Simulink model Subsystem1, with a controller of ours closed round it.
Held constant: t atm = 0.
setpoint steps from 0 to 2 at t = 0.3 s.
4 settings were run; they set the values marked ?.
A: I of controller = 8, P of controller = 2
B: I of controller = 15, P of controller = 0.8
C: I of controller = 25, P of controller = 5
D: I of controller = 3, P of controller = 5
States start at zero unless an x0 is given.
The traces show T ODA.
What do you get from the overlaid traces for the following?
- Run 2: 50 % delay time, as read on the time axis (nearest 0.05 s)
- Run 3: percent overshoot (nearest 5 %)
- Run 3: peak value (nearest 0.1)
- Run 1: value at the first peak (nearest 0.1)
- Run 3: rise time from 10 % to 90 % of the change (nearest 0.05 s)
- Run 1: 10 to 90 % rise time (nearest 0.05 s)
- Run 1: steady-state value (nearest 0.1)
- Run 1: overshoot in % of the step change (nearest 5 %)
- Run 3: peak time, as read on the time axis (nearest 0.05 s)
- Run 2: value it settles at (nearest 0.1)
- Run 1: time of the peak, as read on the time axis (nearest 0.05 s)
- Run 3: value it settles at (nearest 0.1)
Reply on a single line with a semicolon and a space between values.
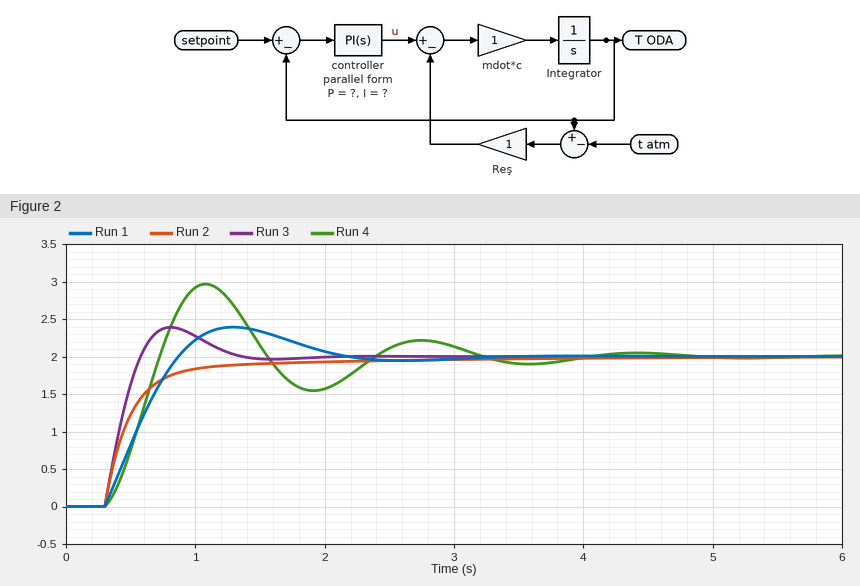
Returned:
0.45 s; 20 %; 2.4; 2.4; 0.20 s; 0.45 s; 2.0; 20 %; 0.80 s; 2.0; 1.30 s; 2.0
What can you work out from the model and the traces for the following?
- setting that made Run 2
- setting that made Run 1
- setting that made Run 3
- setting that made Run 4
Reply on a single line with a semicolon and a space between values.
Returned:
D; A; C; B
